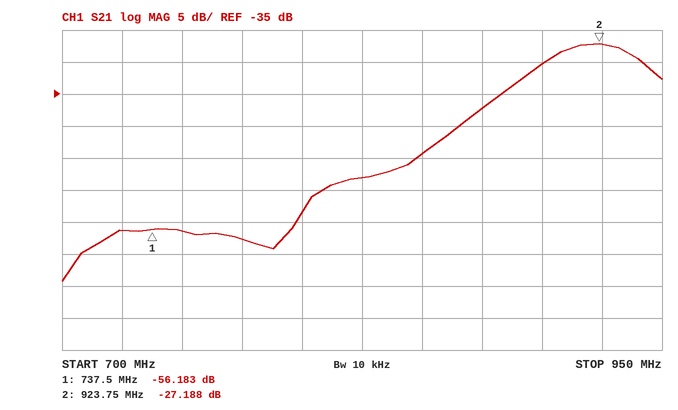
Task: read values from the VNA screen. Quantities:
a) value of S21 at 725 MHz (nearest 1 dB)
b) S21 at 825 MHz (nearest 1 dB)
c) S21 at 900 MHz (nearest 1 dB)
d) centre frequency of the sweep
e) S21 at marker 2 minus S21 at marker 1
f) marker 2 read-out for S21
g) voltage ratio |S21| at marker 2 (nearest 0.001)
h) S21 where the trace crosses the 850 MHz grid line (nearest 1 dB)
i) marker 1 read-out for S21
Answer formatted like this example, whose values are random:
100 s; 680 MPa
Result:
-56 dB; -48 dB; -30 dB; 825 MHz; 28.995 dB; -27.188 dB; 0.044; -44 dB; -56.183 dB
